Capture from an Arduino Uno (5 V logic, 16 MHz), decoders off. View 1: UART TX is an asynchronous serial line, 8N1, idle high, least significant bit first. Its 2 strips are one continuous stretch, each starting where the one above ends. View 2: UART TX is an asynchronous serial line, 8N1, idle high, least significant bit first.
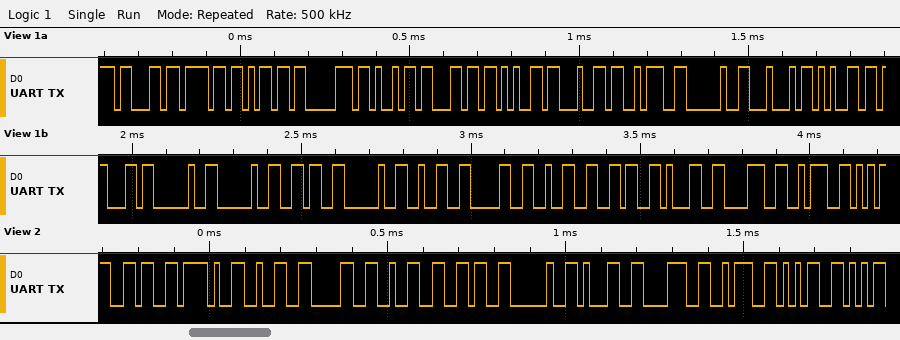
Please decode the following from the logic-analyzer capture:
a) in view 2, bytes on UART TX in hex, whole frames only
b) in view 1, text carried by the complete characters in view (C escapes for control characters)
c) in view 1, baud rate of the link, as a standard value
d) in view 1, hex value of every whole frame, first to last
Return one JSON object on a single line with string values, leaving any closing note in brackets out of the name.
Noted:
{"in view 2, bytes on UART TX in hex, whole frames only": "36 2F 32 30 32 36 20 31 38 3A 35", "in view 1, text carried by the complete characters in view": "\"compiled: Dec  6 202618:\"", "in view 1, baud rate of the link, as a standard value": "57600 baud", "in view 1, hex value of every whole frame, first to last": "63 6F 6D 70 69 6C 65 64 3A 20 44 65 63 20 20 36 20 32 30 32 36 31 38 3A"}
